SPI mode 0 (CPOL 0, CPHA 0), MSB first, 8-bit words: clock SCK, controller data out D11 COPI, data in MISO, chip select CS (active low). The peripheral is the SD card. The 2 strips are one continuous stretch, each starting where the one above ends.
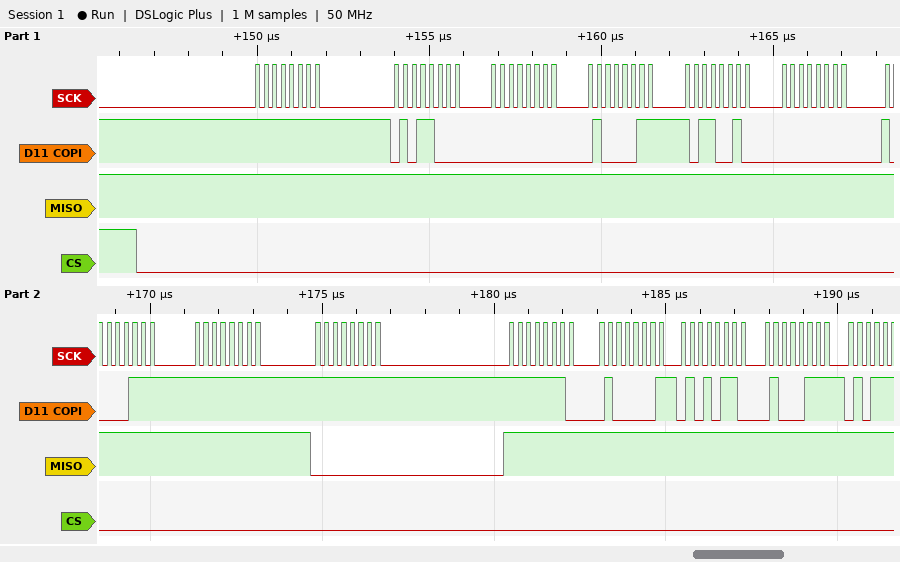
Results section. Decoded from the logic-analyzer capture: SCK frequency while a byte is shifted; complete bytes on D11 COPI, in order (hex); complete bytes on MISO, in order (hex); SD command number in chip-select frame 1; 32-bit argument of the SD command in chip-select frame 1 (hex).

4 MHz
0xFF 0x58 0x00 0x43 0xB2 0x00 0x87 0xFF 0xFF 0xFE 0x41 0x56 0x47
0xFF 0xFF 0xFF 0xFF 0xFF 0xFF 0xFF 0xFF 0x00 0xFF 0xFF 0xFF 0xFF
CMD24
0x0043B200
